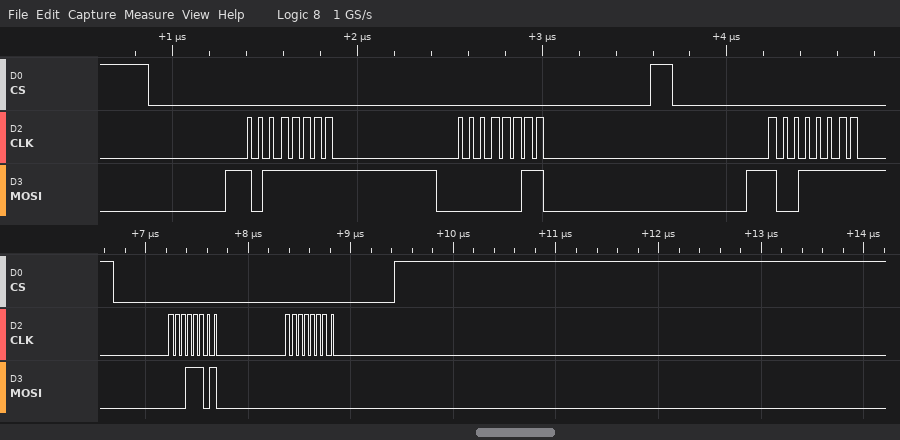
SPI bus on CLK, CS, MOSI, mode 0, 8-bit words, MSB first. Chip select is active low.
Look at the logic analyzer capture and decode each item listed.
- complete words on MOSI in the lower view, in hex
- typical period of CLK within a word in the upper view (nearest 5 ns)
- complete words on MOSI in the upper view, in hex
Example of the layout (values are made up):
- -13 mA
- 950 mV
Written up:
- 1D, 00
- 60 ns
- BF, 03, 9F
